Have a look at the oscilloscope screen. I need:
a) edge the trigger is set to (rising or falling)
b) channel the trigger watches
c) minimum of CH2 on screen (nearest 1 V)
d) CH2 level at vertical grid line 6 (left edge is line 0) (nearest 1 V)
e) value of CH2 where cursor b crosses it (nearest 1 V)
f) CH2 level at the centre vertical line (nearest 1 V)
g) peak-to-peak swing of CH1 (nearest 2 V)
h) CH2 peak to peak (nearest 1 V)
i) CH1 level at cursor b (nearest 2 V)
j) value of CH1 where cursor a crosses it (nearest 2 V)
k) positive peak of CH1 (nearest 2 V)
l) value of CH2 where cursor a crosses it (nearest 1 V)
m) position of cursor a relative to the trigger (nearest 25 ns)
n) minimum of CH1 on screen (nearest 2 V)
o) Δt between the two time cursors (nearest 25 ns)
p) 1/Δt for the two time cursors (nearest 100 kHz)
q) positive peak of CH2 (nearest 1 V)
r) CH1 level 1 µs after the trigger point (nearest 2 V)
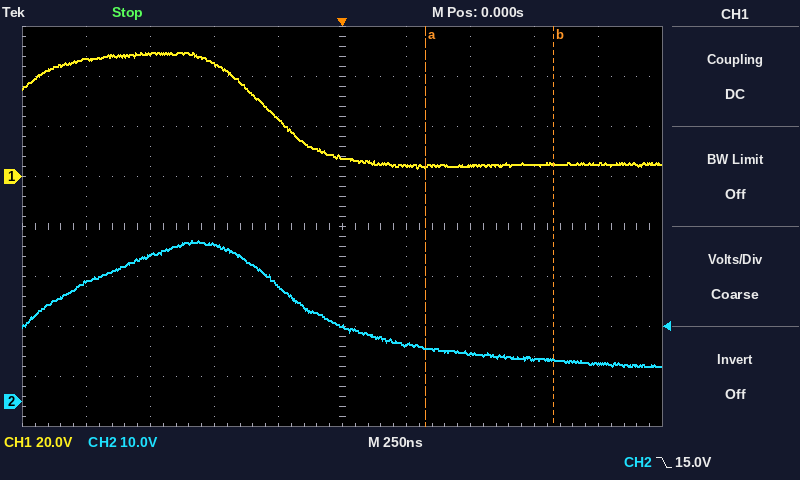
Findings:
falling
CH2
7 V
11 V
8 V
15 V
46 V
25 V
6 V
4 V
50 V
11 V
+325 ns
4 V
500 ns
2.0 MHz
32 V
6 V
